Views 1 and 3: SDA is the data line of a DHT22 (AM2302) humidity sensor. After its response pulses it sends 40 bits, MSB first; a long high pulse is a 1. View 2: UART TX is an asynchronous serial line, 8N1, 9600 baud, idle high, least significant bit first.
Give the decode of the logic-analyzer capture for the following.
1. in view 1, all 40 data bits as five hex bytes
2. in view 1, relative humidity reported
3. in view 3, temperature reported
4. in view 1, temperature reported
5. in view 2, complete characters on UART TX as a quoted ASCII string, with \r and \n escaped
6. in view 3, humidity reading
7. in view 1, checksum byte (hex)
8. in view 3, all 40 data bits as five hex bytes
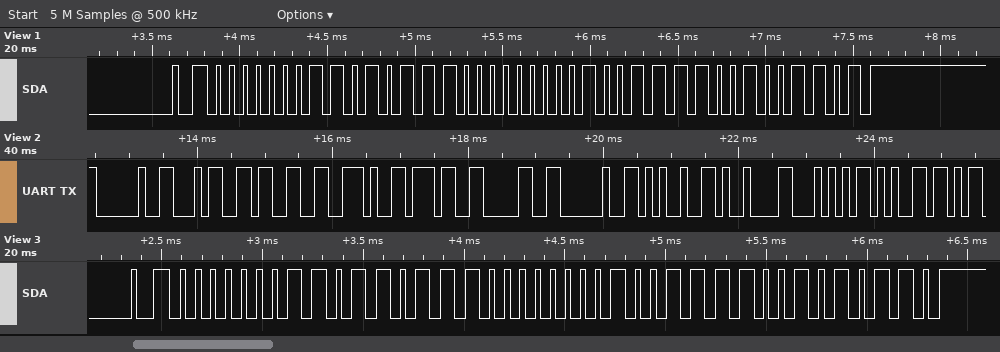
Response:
01 AE 00 9E 4D
43.0 %
15.8 °C
15.8 °C
" 43.70 %\tTe"
43.9 %
0x4D
01 B7 00 9E 56
